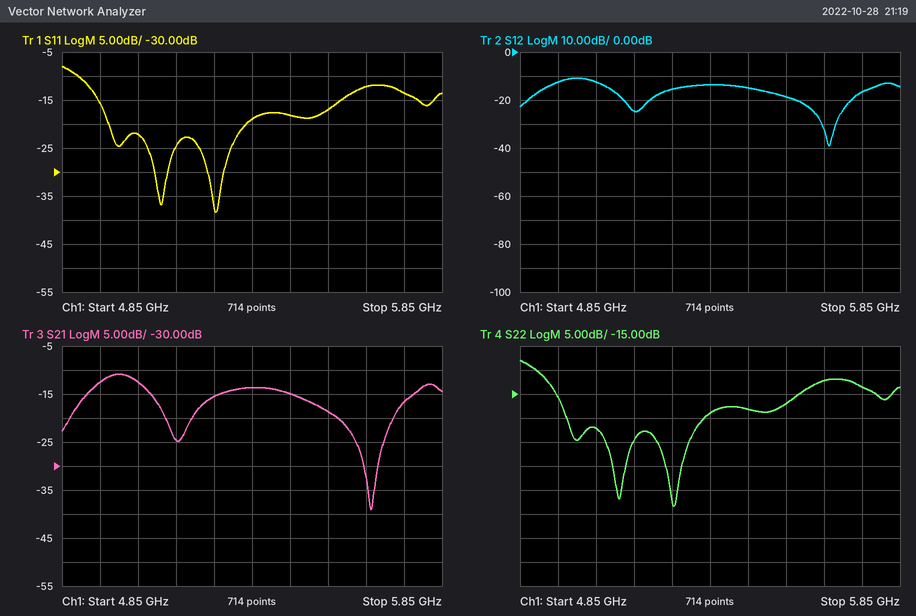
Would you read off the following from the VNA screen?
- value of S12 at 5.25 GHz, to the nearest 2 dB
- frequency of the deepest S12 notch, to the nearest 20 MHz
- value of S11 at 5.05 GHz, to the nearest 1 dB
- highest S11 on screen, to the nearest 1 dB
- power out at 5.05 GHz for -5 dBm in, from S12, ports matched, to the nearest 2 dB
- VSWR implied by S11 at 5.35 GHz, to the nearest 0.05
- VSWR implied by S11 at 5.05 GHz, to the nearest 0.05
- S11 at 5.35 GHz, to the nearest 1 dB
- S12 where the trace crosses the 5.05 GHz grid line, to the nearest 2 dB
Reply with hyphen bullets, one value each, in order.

- -16 dB
- 5.66 GHz
- -22 dB
- -8 dB
- -18 dBm
- 1.25
- 1.15
- -19 dB
- -12 dB
